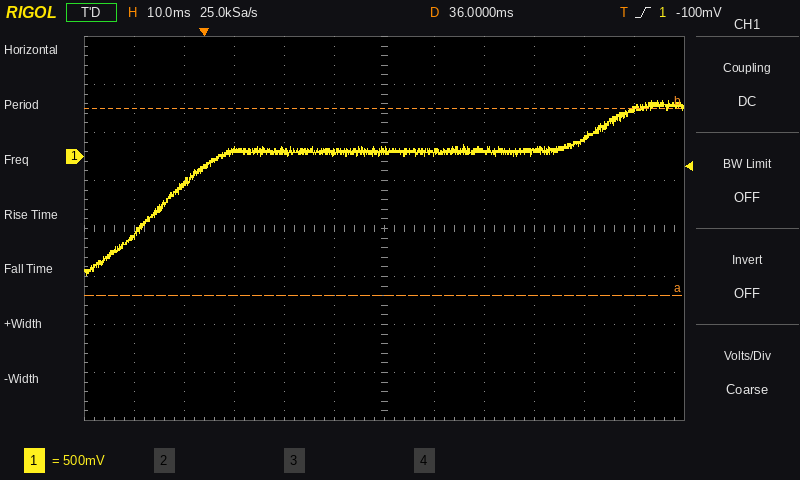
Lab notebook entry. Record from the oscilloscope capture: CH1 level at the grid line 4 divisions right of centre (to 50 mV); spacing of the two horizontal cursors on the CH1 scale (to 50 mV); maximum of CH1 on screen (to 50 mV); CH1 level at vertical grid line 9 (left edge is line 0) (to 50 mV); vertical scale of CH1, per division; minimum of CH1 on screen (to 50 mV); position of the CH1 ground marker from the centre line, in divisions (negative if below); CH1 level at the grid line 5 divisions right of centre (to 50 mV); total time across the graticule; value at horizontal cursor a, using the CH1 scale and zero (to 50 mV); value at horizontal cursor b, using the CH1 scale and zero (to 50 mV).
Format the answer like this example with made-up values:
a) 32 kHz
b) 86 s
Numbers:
a) 200 mV
b) 1.95 V
c) 600 mV
d) 50 mV
e) 500 mV
f) -1.25 V
g) +1.5 div
h) 500 mV
i) 120 ms
j) -1.45 V
k) 500 mV
